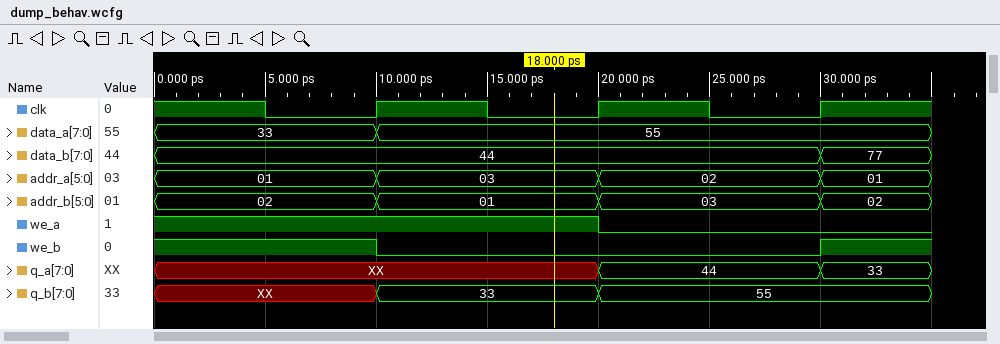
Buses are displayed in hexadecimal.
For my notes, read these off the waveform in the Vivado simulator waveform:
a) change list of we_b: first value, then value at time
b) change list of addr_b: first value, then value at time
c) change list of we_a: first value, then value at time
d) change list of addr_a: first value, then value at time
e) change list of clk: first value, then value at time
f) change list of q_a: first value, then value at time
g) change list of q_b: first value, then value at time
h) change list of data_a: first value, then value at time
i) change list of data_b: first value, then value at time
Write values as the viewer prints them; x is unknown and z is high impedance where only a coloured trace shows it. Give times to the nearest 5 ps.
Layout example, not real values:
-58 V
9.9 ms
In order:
1, 0 at 10 ps, 1 at 30 ps
02, 01 at 10 ps, 03 at 20 ps, 02 at 30 ps
1, 0 at 20 ps
01, 03 at 10 ps, 02 at 20 ps, 01 at 30 ps
1, 0 at 5 ps, 1 at 10 ps, 0 at 15 ps, 1 at 20 ps, 0 at 25 ps, 1 at 30 ps
XX, 44 at 20 ps, 33 at 30 ps
XX, 33 at 10 ps, 55 at 20 ps
33, 55 at 10 ps
44, 77 at 30 ps
